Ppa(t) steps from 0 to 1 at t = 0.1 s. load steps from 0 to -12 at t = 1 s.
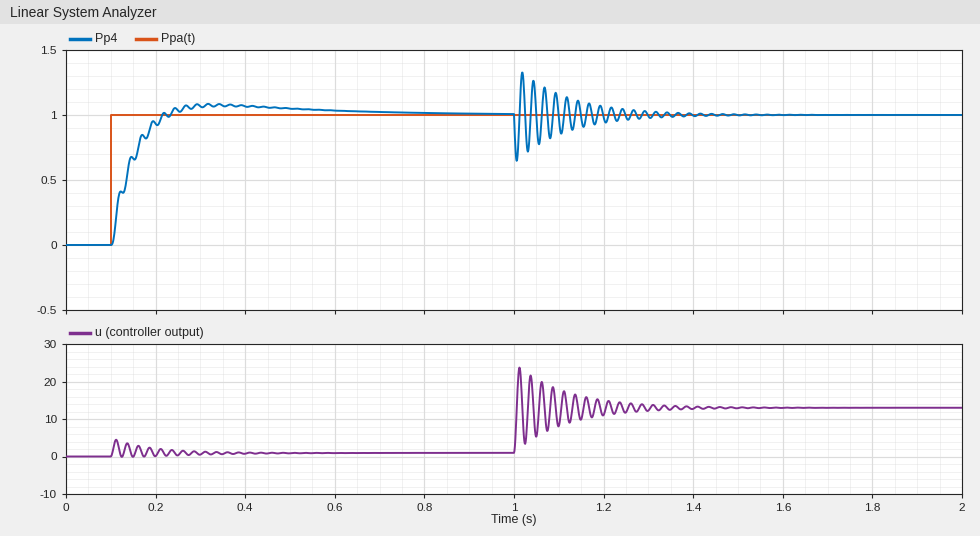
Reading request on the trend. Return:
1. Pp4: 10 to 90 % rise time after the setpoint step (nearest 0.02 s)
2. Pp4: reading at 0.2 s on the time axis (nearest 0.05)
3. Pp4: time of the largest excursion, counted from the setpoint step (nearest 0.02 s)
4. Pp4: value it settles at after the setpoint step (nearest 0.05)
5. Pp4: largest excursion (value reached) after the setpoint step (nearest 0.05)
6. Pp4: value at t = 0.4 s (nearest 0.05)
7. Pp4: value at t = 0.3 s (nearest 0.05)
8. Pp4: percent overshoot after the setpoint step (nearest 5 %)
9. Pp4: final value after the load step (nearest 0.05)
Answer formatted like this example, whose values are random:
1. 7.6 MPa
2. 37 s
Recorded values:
1. 0.08 s
2. 0.95
3. 0.22 s
4. 1.00
5. 1.10
6. 1.05
7. 1.05
8. 10 %
9. 1.00
